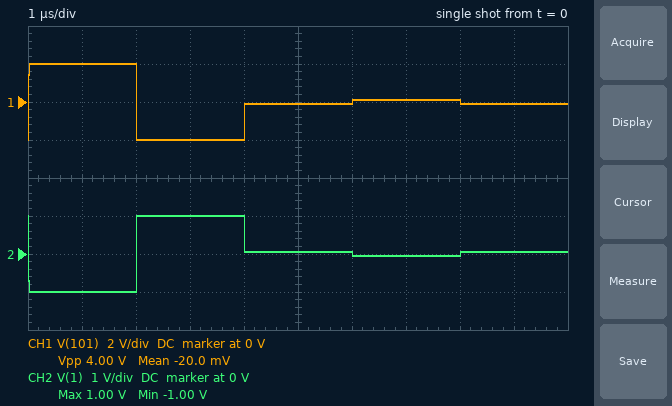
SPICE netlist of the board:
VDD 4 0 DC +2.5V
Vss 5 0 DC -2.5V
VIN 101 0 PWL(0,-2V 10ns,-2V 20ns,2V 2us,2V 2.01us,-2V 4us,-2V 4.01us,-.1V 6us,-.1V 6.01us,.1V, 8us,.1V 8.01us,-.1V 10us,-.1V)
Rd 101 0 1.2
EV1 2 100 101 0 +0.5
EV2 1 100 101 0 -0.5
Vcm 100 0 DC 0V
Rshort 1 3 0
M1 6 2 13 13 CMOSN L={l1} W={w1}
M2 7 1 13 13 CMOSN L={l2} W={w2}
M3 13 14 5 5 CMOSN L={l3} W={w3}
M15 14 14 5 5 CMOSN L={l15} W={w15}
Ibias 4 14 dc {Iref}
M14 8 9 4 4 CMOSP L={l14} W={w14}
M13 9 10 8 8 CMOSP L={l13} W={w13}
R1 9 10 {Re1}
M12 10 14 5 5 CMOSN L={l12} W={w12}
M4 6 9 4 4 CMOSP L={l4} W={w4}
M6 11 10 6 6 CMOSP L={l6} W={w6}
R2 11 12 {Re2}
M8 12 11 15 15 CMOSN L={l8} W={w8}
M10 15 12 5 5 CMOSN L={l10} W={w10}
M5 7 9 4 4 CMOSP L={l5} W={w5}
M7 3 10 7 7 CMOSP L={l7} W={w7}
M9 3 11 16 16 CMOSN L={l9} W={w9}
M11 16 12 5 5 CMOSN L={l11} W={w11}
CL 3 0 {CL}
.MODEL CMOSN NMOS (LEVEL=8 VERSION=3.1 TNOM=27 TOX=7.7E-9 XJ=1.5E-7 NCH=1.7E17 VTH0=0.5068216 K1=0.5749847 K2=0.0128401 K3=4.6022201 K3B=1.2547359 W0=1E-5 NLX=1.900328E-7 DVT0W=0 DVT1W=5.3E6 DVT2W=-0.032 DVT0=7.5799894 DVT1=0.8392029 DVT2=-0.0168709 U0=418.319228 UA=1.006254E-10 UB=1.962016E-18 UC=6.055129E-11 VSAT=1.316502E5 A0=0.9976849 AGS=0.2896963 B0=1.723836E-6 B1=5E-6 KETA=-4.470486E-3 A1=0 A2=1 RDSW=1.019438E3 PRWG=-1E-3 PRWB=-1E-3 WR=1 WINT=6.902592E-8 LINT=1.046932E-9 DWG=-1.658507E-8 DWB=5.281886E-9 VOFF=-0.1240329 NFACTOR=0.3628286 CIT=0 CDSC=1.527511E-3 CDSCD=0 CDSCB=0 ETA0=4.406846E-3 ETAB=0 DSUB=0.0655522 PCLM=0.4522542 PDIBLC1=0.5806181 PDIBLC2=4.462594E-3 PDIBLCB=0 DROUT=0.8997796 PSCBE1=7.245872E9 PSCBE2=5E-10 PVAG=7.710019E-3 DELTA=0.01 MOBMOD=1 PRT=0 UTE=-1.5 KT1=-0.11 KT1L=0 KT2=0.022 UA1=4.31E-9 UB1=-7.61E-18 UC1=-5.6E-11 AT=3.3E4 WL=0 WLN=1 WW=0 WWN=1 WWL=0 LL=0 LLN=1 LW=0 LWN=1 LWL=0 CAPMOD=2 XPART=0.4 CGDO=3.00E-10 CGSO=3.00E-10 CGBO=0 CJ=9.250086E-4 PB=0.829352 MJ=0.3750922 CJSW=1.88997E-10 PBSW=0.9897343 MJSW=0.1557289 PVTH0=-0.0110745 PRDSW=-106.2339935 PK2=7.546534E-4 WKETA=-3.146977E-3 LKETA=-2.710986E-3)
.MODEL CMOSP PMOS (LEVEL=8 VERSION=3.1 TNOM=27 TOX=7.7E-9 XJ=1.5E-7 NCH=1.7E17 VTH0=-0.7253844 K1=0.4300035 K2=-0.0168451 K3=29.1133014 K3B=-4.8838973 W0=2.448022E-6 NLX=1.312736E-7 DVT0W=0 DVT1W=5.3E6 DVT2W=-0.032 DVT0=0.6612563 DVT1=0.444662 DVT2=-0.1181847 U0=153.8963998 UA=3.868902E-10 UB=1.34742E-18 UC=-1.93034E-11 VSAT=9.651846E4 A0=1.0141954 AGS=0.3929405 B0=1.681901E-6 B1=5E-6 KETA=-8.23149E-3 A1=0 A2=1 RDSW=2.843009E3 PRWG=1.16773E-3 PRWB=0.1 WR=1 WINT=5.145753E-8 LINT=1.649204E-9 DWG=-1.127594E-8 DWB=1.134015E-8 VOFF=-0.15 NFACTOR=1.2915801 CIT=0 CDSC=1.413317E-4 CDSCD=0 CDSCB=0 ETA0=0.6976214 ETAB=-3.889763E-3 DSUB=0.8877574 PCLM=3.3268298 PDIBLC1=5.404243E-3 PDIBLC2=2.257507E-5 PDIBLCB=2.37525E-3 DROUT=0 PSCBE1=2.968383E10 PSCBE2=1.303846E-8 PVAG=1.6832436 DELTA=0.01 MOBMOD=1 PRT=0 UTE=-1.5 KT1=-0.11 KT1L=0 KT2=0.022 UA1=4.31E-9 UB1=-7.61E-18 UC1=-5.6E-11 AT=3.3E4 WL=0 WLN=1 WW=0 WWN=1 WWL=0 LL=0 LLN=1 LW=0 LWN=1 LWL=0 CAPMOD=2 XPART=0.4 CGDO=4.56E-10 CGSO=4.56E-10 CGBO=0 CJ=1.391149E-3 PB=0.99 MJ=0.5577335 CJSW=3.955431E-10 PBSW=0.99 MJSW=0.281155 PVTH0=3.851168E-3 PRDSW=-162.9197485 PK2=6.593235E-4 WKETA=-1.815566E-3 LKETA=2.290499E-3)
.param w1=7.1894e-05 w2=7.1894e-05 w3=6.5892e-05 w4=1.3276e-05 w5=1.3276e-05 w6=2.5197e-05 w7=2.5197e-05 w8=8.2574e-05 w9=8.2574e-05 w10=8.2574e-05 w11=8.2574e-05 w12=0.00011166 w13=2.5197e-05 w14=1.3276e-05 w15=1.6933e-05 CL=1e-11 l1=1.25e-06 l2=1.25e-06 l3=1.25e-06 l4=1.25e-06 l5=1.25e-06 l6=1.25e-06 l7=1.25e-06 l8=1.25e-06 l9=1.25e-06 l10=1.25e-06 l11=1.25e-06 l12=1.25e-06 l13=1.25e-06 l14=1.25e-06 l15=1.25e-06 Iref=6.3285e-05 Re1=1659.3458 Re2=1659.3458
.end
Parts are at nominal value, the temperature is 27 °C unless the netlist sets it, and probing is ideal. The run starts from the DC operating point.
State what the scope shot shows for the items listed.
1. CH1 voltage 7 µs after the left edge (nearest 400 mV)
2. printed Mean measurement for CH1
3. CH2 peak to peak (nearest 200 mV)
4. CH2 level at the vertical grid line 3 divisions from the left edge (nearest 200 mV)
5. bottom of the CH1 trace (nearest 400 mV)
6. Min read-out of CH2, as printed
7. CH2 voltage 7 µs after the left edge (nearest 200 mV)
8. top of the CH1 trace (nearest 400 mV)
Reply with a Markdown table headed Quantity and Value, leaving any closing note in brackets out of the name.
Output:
| Quantity | Value |
|---|---|
| CH1 voltage 7 µs after the left edge | 0 V |
| printed Mean measurement for CH1 | -20.0 mV |
| CH2 peak to peak | 2.0 V |
| CH2 level at the vertical grid line 3 divisions from the left edge | 1.0 V |
| bottom of the CH1 trace | -2.0 V |
| Min read-out of CH2, as printed | -1.00 V |
| CH2 voltage 7 µs after the left edge | 0 V |
| top of the CH1 trace | 2.0 V |
